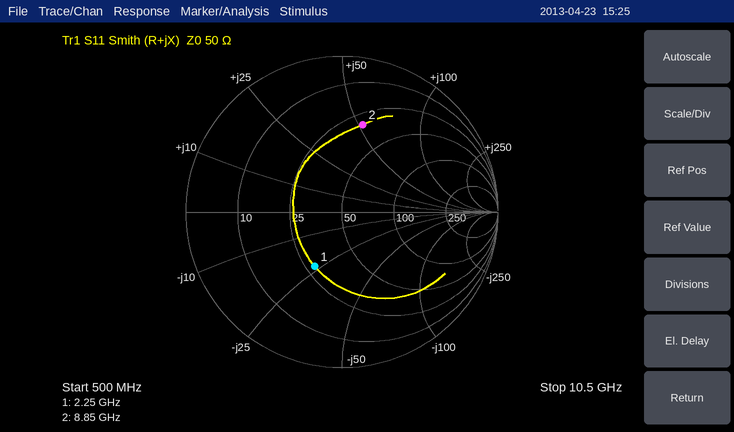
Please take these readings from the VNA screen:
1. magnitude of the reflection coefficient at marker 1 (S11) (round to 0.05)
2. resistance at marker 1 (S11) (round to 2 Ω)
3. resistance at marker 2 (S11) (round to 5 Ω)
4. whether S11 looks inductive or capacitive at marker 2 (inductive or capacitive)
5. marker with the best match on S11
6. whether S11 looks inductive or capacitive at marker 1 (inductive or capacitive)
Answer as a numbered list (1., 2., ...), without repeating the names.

1. 0.40
2. 28 Ω
3. 30 Ω
4. inductive
5. marker 1
6. capacitive
